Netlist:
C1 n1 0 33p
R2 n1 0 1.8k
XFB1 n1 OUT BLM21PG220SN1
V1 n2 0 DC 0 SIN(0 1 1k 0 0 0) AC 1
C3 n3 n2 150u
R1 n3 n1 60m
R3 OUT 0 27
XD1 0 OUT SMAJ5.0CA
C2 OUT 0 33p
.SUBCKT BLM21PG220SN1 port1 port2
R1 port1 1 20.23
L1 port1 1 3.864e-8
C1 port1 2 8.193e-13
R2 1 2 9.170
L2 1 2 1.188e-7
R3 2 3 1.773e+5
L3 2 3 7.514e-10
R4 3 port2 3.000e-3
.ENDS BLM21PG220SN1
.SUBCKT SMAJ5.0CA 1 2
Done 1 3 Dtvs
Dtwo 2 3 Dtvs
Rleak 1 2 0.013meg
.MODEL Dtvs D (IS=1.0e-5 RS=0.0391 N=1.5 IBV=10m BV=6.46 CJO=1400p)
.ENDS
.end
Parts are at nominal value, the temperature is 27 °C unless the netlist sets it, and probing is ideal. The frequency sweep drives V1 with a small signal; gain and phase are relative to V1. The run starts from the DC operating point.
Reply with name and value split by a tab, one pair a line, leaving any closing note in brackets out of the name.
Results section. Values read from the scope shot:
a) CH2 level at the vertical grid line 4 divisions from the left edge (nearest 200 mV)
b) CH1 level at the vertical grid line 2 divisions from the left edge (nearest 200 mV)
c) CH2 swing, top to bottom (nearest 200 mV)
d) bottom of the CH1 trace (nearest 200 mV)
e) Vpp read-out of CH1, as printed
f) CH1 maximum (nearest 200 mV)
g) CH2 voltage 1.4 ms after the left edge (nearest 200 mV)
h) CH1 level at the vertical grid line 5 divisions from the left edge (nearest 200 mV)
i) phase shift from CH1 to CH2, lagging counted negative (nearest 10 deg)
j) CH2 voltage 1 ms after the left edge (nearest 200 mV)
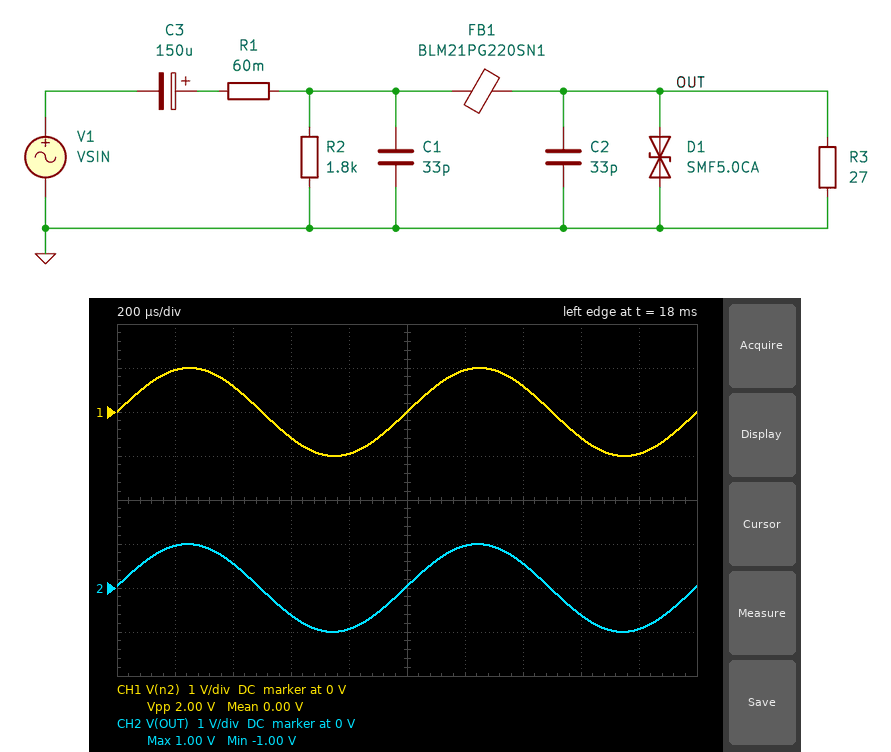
CH2 level at the vertical grid line 4 divisions from the left edge	-1.0 V
CH1 level at the vertical grid line 2 divisions from the left edge	600 mV
CH2 swing, top to bottom	2.0 V
bottom of the CH1 trace	-1.0 V
Vpp read-out of CH1, as printed	2.00 V
CH1 maximum	1.0 V
CH2 voltage 1.4 ms after the left edge	600 mV
CH1 level at the vertical grid line 5 divisions from the left edge	0 V
phase shift from CH1 to CH2, lagging counted negative	0 deg
CH2 voltage 1 ms after the left edge	0 V
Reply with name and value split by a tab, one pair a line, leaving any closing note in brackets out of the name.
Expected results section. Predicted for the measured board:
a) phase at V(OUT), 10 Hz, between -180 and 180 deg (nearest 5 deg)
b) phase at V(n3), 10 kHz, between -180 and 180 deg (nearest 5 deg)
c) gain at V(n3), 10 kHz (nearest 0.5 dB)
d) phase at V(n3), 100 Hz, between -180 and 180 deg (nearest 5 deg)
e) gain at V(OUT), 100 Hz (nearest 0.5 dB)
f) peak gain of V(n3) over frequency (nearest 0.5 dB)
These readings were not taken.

phase at V(OUT), 10 Hz, between -180 and 180 deg	75 deg
phase at V(n3), 10 kHz, between -180 and 180 deg	0 deg
gain at V(n3), 10 kHz	0 dB
phase at V(n3), 100 Hz, between -180 and 180 deg	20 deg
gain at V(OUT), 100 Hz	-0.5 dB
peak gain of V(n3) over frequency	0 dB
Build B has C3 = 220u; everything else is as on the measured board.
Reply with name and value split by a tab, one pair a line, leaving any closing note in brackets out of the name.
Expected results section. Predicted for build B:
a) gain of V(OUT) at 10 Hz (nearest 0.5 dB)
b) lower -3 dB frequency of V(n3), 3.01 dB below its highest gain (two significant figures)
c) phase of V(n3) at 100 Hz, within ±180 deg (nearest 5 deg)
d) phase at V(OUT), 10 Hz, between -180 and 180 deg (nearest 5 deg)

gain of V(OUT) at 10 Hz	-9.5 dB
lower -3 dB frequency of V(n3), 3.01 dB below its highest gain	27 Hz
phase of V(n3) at 100 Hz, within ±180 deg	15 deg
phase at V(OUT), 10 Hz, between -180 and 180 deg	70 deg
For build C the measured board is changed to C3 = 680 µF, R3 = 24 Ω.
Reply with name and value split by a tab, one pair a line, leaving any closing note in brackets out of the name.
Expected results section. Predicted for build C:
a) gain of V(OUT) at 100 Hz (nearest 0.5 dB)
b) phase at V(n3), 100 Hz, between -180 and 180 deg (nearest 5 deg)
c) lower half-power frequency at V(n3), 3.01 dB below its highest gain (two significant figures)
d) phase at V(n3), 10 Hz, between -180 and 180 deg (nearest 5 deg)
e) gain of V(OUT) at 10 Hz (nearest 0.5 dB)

gain of V(OUT) at 100 Hz	0 dB
phase at V(n3), 100 Hz, between -180 and 180 deg	5 deg
lower half-power frequency at V(n3), 3.01 dB below its highest gain	9.9 Hz
phase at V(n3), 10 Hz, between -180 and 180 deg	45 deg
gain of V(OUT) at 10 Hz	-3.0 dB
